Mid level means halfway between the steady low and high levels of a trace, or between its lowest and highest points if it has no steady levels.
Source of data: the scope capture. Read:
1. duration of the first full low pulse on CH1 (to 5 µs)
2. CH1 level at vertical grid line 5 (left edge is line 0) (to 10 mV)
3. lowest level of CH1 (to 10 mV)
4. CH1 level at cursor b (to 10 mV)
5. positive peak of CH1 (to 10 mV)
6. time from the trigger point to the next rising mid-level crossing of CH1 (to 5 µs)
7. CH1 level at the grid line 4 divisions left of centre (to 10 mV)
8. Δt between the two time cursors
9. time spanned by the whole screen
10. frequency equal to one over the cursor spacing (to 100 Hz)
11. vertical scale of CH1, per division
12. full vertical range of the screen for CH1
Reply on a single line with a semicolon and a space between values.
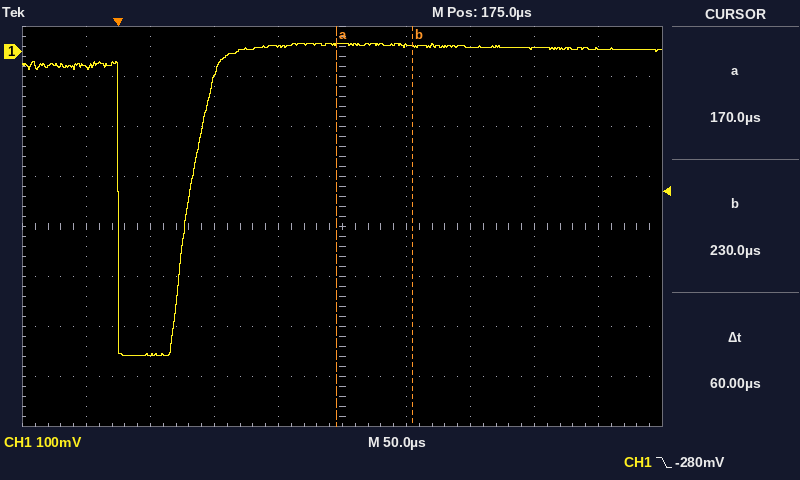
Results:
55 µs; 20 mV; -610 mV; 10 mV; 20 mV; 55 µs; -30 mV; 60 µs; 500 µs; 16.7 kHz; 100 mV; 800 mV
